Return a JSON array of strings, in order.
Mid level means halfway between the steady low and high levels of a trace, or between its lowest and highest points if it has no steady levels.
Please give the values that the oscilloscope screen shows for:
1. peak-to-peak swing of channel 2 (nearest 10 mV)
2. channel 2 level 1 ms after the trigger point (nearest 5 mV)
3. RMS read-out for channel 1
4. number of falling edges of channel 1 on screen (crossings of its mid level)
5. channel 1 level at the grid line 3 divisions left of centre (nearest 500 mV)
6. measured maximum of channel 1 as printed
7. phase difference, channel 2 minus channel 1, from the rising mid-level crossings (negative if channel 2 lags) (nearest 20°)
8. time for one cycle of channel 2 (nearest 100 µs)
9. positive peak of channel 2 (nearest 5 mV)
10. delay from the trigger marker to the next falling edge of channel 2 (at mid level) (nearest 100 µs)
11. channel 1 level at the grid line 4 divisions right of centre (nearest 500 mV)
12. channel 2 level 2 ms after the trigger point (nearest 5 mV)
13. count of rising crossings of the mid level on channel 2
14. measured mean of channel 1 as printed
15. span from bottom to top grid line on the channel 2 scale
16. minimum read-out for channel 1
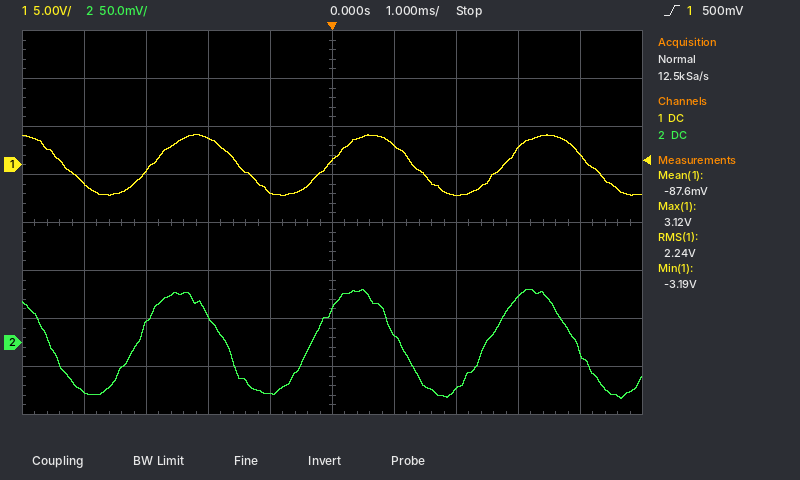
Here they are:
["110 mV", "10 mV", "2.24 V", "4", "-500 mV", "3.12 V", "+40°", "2.8 ms", "55 mV", "1.1 ms", "1.0 V", "-50 mV", "3", "-87.6 mV", "400 mV", "-3.19 V"]
